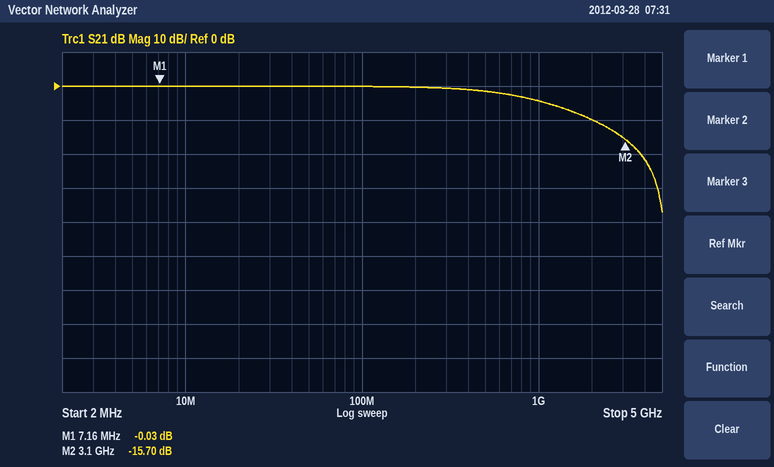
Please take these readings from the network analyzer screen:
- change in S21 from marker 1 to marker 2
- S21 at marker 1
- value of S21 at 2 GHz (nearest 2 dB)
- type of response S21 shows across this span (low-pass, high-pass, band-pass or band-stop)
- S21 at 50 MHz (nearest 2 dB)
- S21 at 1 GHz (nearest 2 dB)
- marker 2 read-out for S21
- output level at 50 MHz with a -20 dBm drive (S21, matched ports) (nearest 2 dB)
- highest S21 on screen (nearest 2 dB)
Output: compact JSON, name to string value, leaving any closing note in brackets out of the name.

{"change in S21 from marker 1 to marker 2": "-15.67 dB", "S21 at marker 1": "-0.03 dB", "value of S21 at 2 GHz": "-10 dB", "type of response S21 shows across this span": "low-pass", "S21 at 50 MHz": "0 dB", "S21 at 1 GHz": "-4 dB", "marker 2 read-out for S21": "-15.70 dB", "output level at 50 MHz with a -20 dBm drive (S21, matched ports)": "-20 dBm", "highest S21 on screen": "0 dB"}
